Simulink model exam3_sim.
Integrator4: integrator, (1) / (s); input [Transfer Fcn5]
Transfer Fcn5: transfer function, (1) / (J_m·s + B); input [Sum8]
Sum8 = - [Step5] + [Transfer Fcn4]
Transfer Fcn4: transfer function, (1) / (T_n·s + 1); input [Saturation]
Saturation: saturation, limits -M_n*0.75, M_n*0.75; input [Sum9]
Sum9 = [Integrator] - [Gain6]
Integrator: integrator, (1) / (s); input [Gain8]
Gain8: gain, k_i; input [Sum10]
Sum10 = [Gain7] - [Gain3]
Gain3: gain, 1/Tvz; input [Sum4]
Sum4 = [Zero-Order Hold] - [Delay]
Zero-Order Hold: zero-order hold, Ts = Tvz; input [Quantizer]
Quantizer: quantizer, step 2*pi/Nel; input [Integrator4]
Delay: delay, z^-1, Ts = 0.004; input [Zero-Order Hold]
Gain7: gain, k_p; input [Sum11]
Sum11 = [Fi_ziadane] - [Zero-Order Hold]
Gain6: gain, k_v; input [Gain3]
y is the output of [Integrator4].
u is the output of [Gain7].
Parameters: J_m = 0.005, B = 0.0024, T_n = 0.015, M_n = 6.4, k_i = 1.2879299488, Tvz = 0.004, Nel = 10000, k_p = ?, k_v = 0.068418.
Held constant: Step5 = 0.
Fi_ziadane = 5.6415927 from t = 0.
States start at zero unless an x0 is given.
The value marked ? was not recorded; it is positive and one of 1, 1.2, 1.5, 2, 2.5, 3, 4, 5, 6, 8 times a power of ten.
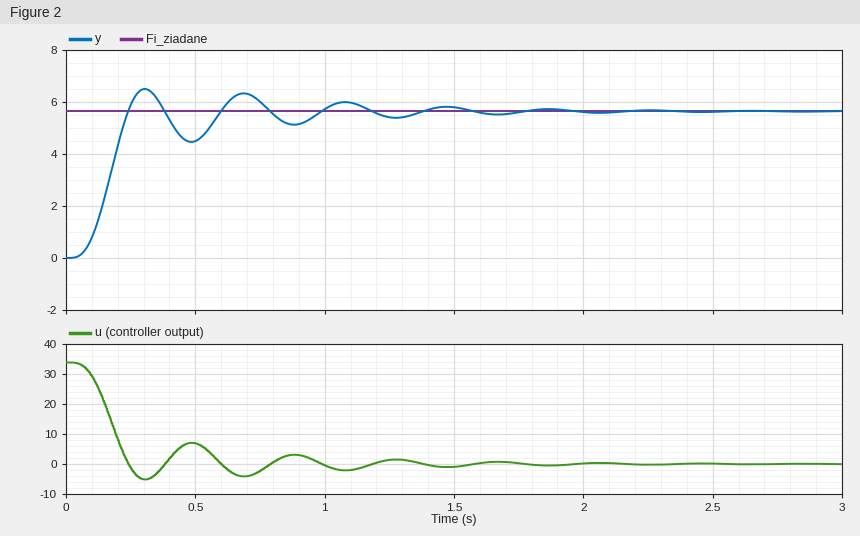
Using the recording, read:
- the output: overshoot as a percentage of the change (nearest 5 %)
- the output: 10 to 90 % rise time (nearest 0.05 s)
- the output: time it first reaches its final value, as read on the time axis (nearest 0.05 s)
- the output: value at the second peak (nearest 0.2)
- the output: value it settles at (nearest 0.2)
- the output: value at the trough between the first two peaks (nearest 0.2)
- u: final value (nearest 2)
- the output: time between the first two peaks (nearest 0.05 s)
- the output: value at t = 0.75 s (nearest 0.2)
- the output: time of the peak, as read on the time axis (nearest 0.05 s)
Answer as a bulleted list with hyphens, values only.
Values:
- 15 %
- 0.15 s
- 0.25 s
- 6.4
- 5.6
- 4.4
- 0
- 0.40 s
- 6.0
- 0.30 s
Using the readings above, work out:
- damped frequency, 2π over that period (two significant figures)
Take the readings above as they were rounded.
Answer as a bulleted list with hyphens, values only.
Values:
- 16 rad/s
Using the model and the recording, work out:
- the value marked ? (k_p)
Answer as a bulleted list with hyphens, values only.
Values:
- 6
